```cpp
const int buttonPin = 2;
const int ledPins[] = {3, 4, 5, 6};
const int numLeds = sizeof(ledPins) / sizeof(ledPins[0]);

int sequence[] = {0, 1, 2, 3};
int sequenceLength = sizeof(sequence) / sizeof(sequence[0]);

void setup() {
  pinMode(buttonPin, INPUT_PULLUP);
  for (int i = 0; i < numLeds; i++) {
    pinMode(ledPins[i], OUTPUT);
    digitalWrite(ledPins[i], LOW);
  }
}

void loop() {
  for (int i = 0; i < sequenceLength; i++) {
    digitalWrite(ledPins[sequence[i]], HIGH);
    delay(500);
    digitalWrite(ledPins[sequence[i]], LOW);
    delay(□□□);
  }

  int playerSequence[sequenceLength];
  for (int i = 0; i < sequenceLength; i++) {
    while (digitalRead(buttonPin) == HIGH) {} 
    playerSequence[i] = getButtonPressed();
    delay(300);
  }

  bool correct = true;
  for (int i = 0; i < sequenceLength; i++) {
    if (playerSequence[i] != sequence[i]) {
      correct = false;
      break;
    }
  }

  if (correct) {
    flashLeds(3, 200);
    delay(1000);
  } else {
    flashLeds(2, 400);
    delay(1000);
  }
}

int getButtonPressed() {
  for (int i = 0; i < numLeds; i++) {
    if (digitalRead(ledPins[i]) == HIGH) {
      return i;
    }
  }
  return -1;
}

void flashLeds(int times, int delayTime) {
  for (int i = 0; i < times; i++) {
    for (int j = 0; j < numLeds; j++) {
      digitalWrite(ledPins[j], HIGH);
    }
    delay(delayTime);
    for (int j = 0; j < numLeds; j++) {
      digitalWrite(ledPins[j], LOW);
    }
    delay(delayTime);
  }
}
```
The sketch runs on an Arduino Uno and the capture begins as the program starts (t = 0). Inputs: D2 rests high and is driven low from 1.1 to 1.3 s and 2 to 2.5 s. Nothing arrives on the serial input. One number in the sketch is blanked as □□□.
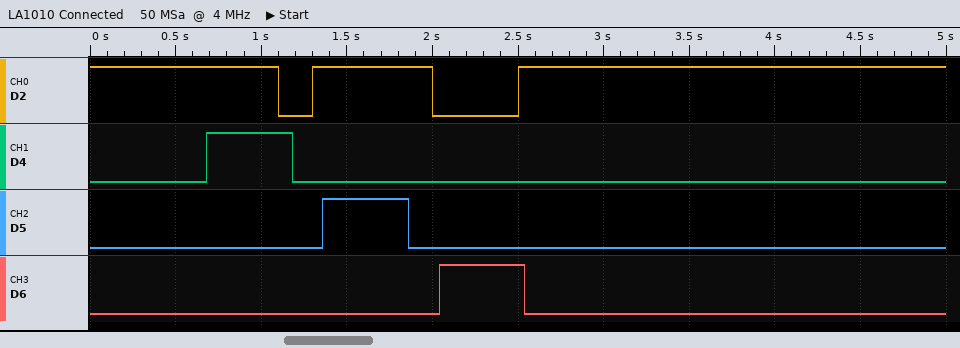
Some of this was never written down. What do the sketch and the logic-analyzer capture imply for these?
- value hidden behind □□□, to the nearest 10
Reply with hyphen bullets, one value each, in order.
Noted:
- 180
